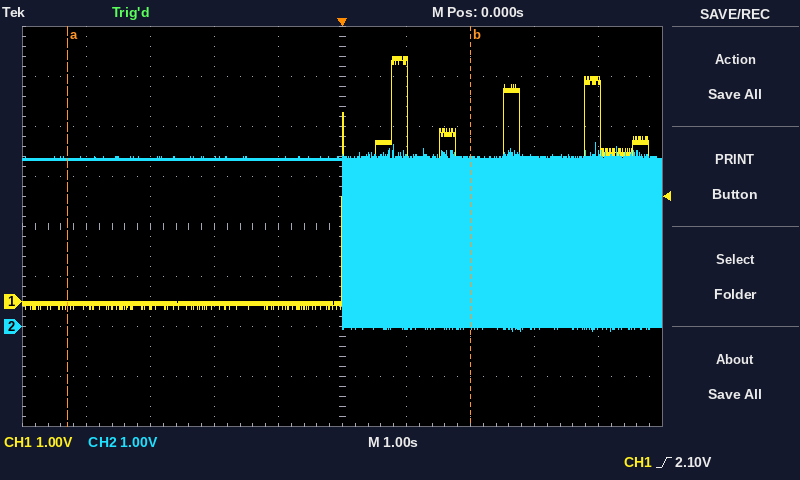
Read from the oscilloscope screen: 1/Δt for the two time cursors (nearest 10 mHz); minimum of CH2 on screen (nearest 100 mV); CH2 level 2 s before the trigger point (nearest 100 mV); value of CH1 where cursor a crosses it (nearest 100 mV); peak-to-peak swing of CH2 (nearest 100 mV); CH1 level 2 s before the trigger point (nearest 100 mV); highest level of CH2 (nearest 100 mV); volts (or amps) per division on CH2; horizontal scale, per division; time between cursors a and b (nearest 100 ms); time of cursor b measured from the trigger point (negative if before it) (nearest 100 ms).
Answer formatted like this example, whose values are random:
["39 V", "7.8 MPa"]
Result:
["160 mHz", "-100 mV", "3.4 V", "-100 mV", "3.8 V", "-100 mV", "3.7 V", "1 V", "1 s", "6.3 s", "+2.0 s"]
